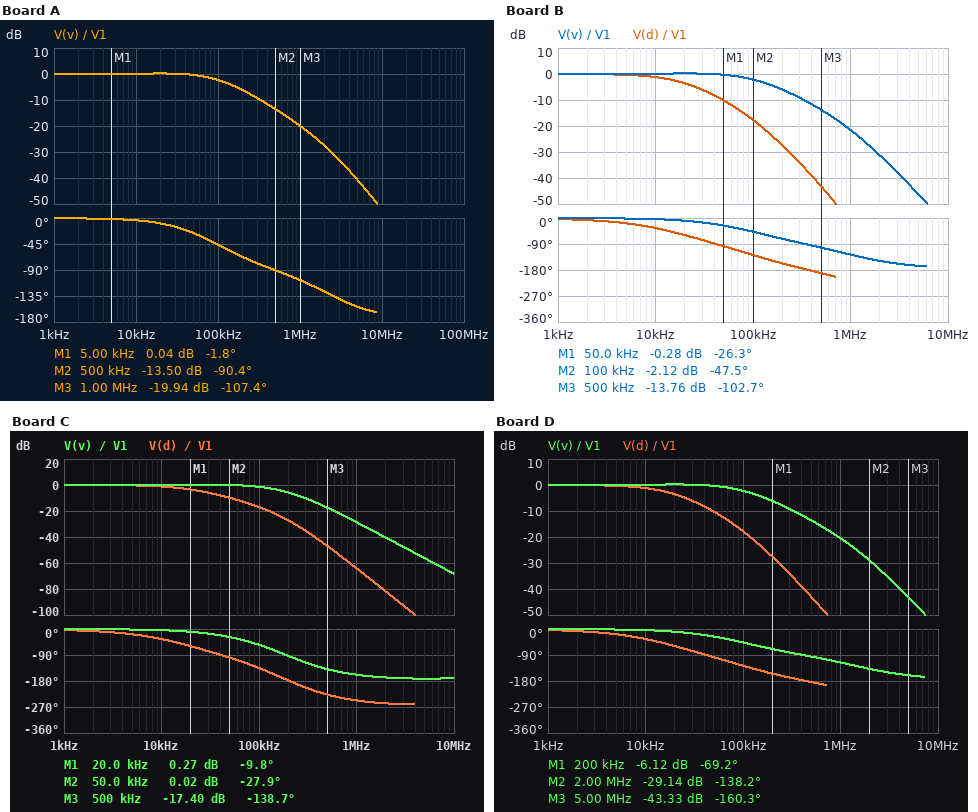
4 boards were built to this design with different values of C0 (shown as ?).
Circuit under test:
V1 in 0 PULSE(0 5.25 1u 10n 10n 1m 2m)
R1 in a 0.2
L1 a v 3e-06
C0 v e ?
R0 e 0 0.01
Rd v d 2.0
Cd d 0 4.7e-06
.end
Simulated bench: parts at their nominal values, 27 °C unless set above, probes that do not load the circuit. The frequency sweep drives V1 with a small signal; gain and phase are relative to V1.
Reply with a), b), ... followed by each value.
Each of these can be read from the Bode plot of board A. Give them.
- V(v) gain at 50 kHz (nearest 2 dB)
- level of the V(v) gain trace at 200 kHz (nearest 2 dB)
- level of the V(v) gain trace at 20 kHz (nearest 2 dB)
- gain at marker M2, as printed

a) 0 dB
b) -6 dB
c) 0 dB
d) -13.50 dB
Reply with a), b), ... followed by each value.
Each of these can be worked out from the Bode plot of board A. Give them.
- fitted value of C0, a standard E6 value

a) 33 nF
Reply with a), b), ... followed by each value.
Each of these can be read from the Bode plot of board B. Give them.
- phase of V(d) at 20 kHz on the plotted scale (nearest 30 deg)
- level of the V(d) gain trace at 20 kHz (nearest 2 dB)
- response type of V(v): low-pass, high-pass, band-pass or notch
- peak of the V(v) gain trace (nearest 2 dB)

a) -60 deg
b) -4 dB
c) low-pass
d) 0 dB
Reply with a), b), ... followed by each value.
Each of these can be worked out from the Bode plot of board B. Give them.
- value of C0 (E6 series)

a) 68 nF
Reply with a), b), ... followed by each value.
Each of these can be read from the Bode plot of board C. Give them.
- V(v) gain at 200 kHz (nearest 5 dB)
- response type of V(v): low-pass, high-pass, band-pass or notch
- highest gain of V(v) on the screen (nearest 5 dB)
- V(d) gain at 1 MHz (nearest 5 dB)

a) -5 dB
b) low-pass
c) 0 dB
d) -65 dB
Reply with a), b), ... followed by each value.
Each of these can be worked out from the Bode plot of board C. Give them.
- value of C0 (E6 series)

a) 220 nF
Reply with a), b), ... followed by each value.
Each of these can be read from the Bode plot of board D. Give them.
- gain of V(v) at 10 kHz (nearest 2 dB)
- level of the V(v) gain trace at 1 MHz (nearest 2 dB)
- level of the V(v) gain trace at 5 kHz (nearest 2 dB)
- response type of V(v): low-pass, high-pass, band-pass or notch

a) 0 dB
b) -20 dB
c) 0 dB
d) low-pass
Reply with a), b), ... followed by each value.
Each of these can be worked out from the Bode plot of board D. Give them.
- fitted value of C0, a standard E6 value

a) 47 nF
